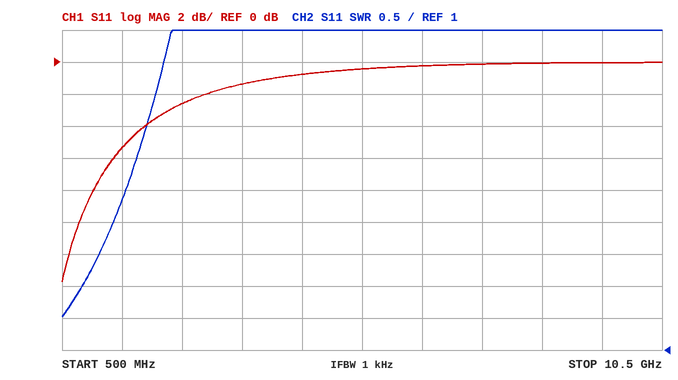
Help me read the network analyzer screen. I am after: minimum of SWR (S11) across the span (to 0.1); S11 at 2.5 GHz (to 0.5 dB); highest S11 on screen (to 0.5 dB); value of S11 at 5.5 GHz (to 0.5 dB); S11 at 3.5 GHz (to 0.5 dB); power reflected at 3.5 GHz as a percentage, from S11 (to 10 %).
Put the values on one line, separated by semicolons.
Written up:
1.5; -2.5 dB; 0.0 dB; -0.5 dB; -1.5 dB; 70 %
